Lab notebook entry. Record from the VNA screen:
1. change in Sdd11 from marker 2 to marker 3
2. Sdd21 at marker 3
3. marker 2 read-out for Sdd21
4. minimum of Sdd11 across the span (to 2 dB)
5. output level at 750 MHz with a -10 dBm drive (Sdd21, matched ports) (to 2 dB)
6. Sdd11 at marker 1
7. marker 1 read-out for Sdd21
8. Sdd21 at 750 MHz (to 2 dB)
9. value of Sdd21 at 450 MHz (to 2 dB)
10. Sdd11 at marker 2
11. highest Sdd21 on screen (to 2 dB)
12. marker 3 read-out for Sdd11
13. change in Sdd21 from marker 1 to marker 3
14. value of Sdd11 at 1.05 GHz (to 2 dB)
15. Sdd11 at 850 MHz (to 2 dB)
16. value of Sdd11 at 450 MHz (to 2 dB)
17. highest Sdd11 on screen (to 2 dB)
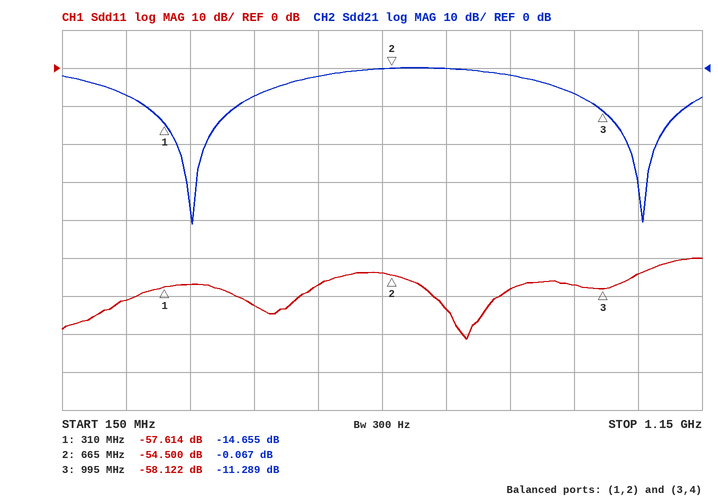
-3.622 dB
-11.289 dB
-0.067 dB
-72 dB
-10 dBm
-57.614 dB
-14.655 dB
0 dB
-8 dB
-54.500 dB
0 dB
-58.122 dB
3.366 dB
-54 dB
-58 dB
-62 dB
-50 dB
